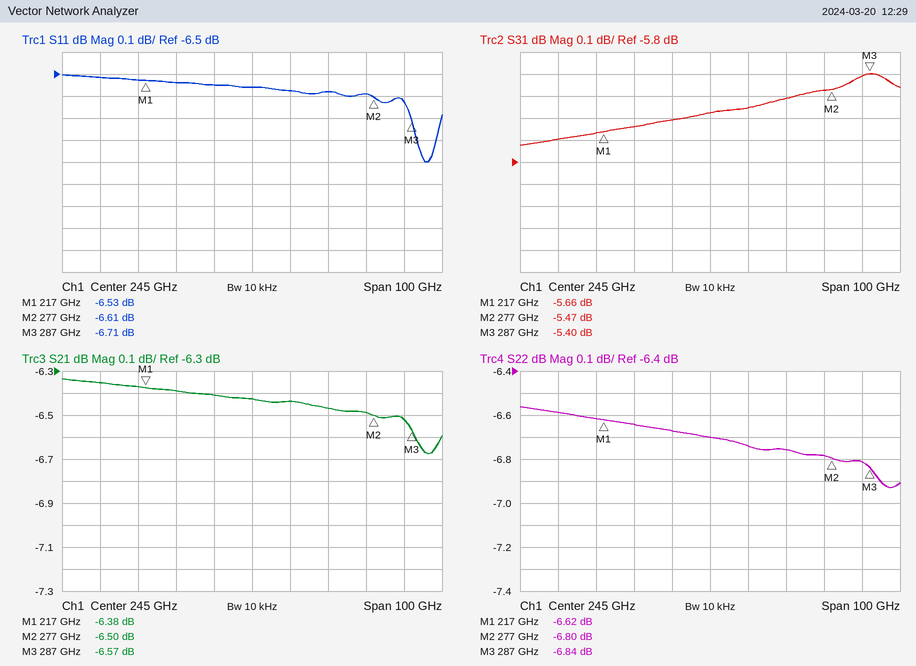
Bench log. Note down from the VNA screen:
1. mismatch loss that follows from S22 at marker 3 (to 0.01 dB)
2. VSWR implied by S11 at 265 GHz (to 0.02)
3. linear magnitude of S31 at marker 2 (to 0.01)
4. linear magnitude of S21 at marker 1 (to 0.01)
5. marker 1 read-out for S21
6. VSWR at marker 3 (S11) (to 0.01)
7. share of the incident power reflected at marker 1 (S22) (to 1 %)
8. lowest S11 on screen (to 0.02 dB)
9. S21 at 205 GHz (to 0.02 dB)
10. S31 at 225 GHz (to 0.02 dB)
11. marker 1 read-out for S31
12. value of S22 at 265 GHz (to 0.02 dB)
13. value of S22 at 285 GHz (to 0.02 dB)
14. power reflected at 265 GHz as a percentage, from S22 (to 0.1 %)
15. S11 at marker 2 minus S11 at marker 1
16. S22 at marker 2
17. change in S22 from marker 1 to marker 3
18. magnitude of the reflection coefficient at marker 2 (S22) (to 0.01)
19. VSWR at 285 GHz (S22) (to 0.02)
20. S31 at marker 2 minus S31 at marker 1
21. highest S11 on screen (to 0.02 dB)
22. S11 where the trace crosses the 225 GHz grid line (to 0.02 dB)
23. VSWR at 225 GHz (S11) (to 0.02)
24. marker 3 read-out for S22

1.01 dB
2.76
0.53
0.48
-6.38 dB
2.72
22 %
-6.90 dB
-6.36 dB
-5.64 dB
-5.66 dB
-6.76 dB
-6.82 dB
21.1 %
-0.08 dB
-6.80 dB
-0.22 dB
0.46
2.68
0.19 dB
-6.50 dB
-6.54 dB
2.78
-6.84 dB
